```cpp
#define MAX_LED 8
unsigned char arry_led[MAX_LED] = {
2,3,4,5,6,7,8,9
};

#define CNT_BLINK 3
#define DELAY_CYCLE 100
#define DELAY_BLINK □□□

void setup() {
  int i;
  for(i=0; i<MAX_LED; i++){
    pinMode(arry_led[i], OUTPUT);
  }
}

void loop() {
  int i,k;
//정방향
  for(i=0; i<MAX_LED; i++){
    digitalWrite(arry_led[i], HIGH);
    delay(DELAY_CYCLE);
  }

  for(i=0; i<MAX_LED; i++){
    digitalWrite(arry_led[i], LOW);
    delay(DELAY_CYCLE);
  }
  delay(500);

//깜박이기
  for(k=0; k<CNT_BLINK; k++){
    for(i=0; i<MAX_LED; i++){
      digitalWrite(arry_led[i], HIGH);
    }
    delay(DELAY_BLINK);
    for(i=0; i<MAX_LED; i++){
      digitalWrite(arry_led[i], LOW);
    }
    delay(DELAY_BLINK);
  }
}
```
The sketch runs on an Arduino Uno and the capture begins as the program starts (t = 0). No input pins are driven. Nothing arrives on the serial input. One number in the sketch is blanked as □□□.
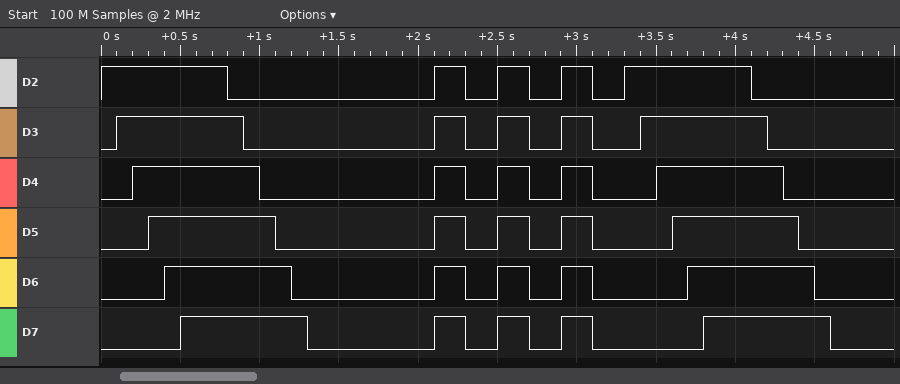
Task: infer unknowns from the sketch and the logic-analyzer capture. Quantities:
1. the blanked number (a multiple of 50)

200
